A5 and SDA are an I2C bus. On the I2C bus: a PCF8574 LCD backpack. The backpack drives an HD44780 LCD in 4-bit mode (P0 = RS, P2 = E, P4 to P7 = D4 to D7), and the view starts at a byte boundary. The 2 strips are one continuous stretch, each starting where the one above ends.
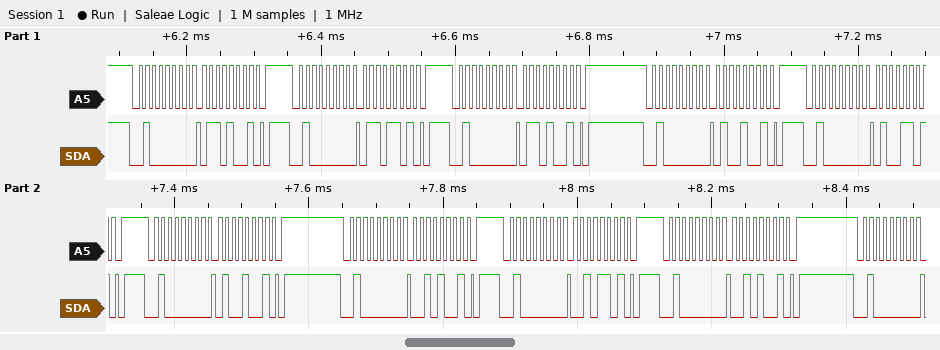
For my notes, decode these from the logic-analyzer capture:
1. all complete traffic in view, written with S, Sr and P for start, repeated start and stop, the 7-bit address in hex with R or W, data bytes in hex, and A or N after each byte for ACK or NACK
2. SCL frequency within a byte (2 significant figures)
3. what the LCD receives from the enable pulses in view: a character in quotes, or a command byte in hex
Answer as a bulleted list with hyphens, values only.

- S 20W A 69 A P S 20W A 6D A P S 20W A 69 A P S 20W A 49 A P S 20W A 4D A P S 20W A 49 A P S 20W A 29 A P S 20W A 2D A P S 20W A 29 A P S 20W A
- 100 kHz
- 'd'
